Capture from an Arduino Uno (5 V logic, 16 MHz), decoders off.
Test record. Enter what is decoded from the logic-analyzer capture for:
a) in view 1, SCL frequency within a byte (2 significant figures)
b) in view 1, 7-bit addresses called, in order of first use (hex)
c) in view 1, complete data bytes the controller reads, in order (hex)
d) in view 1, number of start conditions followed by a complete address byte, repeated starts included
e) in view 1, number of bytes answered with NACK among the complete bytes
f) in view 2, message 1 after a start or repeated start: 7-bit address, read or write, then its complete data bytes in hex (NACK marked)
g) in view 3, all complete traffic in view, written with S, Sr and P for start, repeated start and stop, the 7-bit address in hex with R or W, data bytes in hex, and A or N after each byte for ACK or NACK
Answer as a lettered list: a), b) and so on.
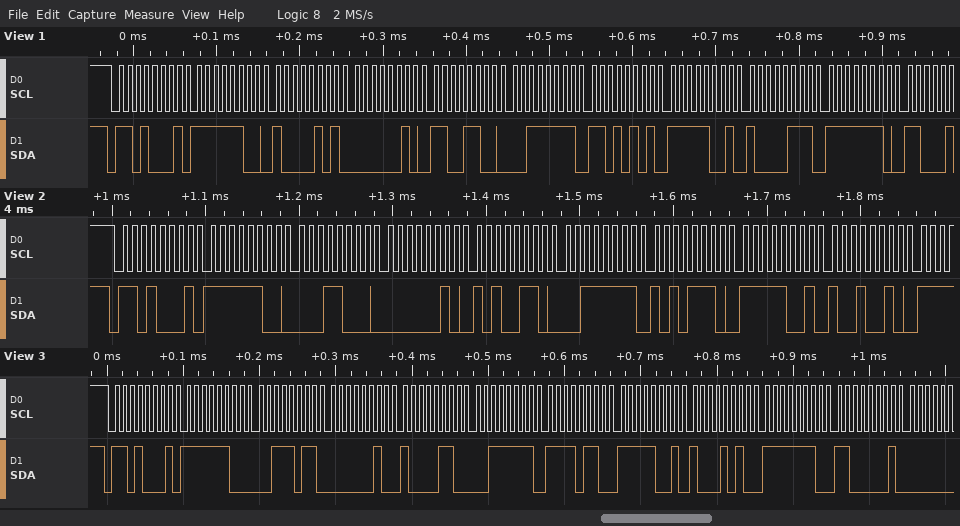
a) 100 kHz
b) 0x68
c) FC 85 02 CC 3F D5 F9 87 FE
d) 1
e) 0
f) 0x68 read: FC 18 02 A6 3F AE F9 92
g) S 68R A FC A 3B A 02 A 86 A 3F A F6 A F9 A 8A A FE A C1 A
